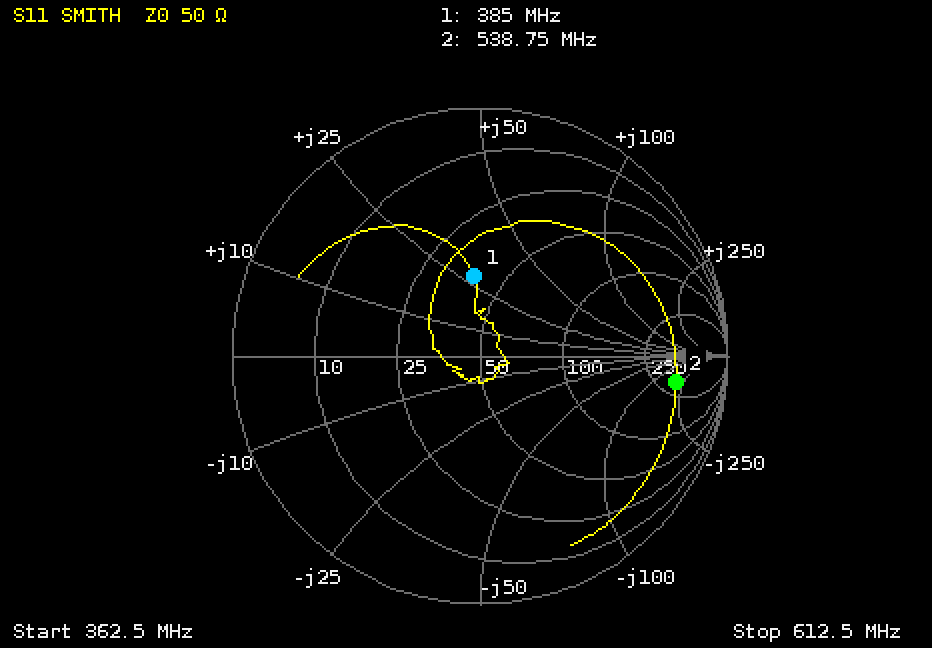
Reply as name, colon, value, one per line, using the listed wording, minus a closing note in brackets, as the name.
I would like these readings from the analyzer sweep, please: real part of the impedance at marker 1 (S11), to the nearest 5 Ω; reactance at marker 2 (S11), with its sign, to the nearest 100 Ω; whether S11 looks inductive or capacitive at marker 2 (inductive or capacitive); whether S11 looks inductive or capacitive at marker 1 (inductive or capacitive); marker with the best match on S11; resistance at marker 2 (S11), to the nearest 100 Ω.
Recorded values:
real part of the impedance at marker 1 (S11), to the nearest 5 Ω: 40 Ω
reactance at marker 2 (S11), with its sign, to the nearest 100 Ω: -200 Ω
whether S11 looks inductive or capacitive at marker 2: capacitive
whether S11 looks inductive or capacitive at marker 1: inductive
marker with the best match on S11: marker 1
resistance at marker 2 (S11), to the nearest 100 Ω: 300 Ω
